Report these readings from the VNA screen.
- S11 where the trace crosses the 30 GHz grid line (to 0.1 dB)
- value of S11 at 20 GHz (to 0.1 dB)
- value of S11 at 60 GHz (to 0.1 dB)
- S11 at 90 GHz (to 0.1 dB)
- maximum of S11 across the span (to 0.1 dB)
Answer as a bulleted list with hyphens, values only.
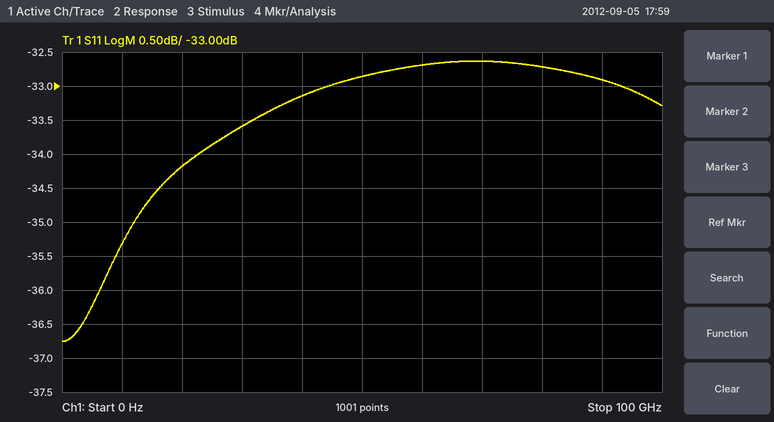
- -33.6 dB
- -34.2 dB
- -32.7 dB
- -32.9 dB
- -32.6 dB
